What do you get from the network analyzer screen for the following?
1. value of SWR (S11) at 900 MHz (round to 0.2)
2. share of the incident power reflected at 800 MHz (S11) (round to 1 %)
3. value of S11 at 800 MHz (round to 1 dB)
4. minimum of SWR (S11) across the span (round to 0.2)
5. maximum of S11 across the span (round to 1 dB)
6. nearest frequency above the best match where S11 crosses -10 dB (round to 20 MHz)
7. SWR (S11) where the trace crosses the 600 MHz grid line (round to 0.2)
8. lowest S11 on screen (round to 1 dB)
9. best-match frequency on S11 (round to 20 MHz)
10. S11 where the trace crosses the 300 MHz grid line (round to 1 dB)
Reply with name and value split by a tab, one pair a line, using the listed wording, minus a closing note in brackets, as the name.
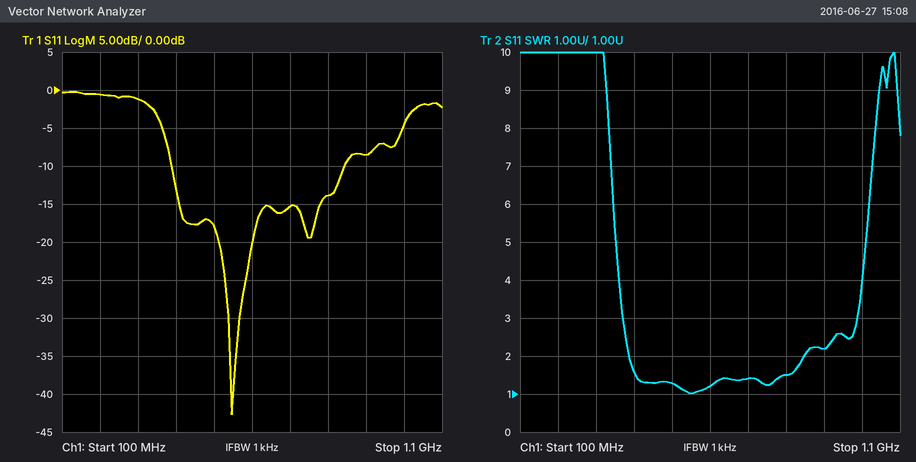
value of SWR (S11) at 900 MHz	2.2
share of the incident power reflected at 800 MHz (S11)	4 %
value of S11 at 800 MHz	-14 dB
minimum of SWR (S11) across the span	1.0
maximum of S11 across the span	0 dB
nearest frequency above the best match where S11 crosses -10 dB	840 MHz
SWR (S11) where the trace crosses the 600 MHz grid line	1.2
lowest S11 on screen	-43 dB
best-match frequency on S11	540 MHz
S11 where the trace crosses the 300 MHz grid line	-1 dB
